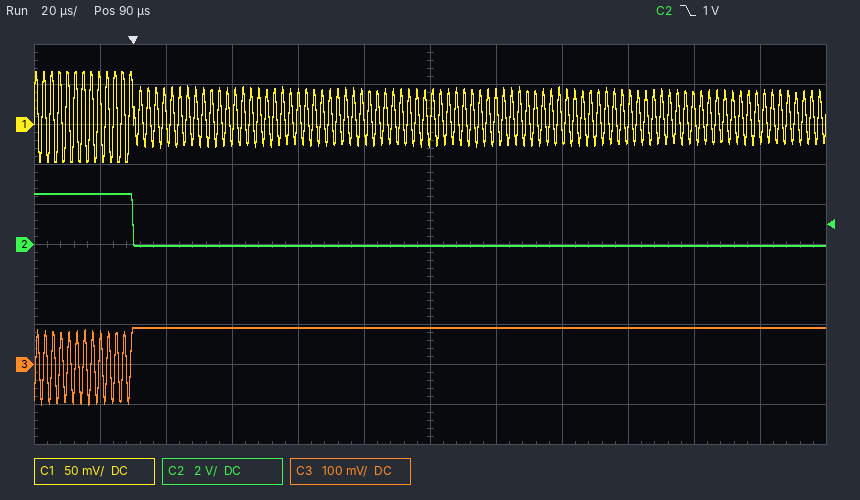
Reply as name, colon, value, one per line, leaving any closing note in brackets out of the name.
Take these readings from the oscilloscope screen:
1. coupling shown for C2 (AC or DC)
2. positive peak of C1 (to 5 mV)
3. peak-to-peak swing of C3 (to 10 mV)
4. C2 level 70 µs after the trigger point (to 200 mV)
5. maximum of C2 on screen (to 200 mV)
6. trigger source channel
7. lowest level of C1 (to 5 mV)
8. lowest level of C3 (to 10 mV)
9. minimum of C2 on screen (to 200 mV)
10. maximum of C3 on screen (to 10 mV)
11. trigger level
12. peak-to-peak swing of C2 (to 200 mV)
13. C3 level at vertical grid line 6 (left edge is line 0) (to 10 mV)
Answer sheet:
coupling shown for C2: DC
positive peak of C1: 65 mV
peak-to-peak swing of C3: 190 mV
C2 level 70 µs after the trigger point: 0.0 V
maximum of C2 on screen: 2.6 V
trigger source channel: C2
lowest level of C1: -45 mV
lowest level of C3: -100 mV
minimum of C2 on screen: 0.0 V
maximum of C3 on screen: 90 mV
trigger level: 1 V
peak-to-peak swing of C2: 2.6 V
C3 level at vertical grid line 6 (left edge is line 0): 90 mV
